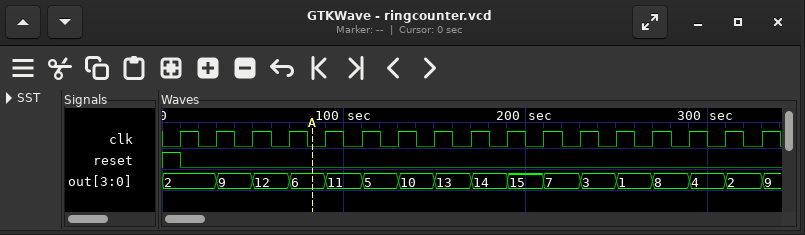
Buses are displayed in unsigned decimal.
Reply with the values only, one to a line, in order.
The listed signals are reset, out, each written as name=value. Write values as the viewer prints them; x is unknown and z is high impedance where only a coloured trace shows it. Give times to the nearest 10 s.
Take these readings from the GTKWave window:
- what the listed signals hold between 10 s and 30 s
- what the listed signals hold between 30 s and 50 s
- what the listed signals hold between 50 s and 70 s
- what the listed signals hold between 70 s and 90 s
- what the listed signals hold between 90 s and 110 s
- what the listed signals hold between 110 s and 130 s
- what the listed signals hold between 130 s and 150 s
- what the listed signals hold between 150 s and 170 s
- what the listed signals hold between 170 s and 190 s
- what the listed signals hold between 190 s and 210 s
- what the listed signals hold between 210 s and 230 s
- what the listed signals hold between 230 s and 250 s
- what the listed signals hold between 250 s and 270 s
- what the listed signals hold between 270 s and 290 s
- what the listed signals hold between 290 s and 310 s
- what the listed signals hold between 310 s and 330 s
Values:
reset=0, out=2
reset=0, out=9
reset=0, out=12
reset=0, out=6
reset=0, out=11
reset=0, out=5
reset=0, out=10
reset=0, out=13
reset=0, out=14
reset=0, out=15
reset=0, out=7
reset=0, out=3
reset=0, out=1
reset=0, out=8
reset=0, out=4
reset=0, out=2
